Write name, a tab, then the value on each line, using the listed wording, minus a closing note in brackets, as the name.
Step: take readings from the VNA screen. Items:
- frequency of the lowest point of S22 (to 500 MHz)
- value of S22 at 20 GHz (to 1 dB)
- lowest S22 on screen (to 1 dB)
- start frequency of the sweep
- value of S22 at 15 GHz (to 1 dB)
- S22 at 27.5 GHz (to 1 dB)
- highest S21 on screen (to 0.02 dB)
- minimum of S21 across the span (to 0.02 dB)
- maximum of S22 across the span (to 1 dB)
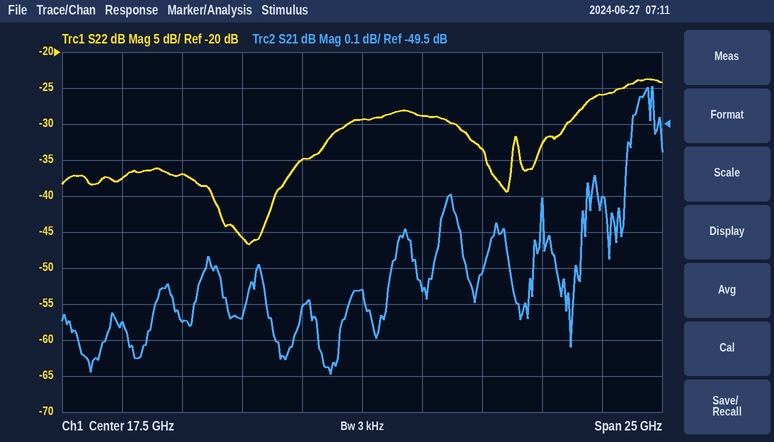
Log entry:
frequency of the lowest point of S22	13.0 GHz
value of S22 at 20 GHz	-29 dB
lowest S22 on screen	-47 dB
start frequency of the sweep	5 GHz
value of S22 at 15 GHz	-35 dB
S22 at 27.5 GHz	-26 dB
highest S21 on screen	-49.40 dB
minimum of S21 across the span	-50.20 dB
maximum of S22 across the span	-24 dB
